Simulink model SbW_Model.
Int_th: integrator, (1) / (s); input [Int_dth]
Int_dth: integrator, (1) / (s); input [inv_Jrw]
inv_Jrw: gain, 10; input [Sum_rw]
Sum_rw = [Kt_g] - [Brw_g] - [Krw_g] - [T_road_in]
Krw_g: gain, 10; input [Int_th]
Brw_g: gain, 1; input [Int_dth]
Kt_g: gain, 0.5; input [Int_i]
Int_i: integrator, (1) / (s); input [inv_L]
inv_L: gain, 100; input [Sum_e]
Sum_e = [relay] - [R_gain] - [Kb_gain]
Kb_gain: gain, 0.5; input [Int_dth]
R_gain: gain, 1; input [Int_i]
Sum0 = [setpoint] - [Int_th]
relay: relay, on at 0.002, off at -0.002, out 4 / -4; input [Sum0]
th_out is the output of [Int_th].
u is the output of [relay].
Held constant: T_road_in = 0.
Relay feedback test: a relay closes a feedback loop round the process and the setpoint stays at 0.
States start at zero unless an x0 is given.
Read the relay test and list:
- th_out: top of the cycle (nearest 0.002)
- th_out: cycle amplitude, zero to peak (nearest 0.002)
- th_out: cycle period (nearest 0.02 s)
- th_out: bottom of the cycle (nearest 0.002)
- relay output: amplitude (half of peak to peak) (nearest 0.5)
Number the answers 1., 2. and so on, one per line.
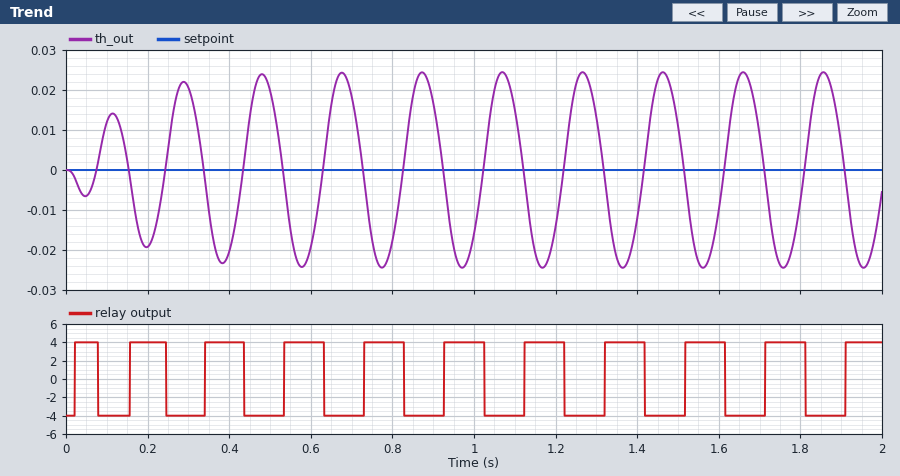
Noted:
1. 0.024
2. 0.024
3. 0.20 s
4. -0.024
5. 4.0
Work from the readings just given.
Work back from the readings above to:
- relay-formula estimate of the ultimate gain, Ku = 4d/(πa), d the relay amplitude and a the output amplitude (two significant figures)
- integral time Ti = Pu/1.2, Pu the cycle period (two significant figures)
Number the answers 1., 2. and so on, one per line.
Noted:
1. 210
2. 0.17 s
